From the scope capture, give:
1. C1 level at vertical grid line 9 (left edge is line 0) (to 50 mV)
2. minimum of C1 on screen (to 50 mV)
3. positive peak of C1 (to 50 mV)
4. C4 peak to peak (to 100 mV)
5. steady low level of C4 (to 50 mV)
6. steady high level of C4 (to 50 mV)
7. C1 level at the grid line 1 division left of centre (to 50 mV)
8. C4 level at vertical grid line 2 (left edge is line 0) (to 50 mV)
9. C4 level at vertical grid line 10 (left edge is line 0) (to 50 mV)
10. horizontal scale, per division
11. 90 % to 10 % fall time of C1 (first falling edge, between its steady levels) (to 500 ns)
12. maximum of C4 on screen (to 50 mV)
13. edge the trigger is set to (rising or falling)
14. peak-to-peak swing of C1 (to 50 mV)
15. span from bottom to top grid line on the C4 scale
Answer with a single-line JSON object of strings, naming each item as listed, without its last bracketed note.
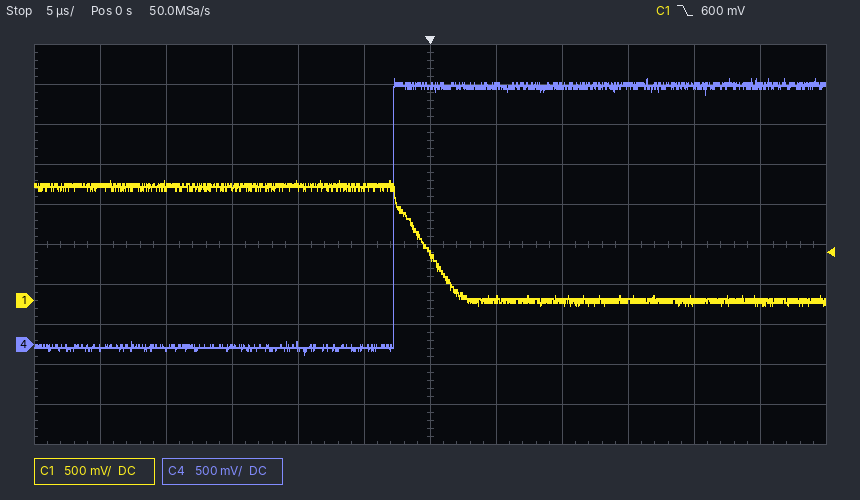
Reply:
{"C1 level at vertical grid line 9 (left edge is line 0)": "0 mV", "minimum of C1 on screen": "-50 mV", "positive peak of C1": "1.50 V", "C4 peak to peak": "3.40 V", "steady low level of C4": "-50 mV", "steady high level of C4": "3.25 V", "C1 level at the grid line 1 division left of centre": "1.40 V", "C4 level at vertical grid line 2 (left edge is line 0)": "-50 mV", "C4 level at vertical grid line 10 (left edge is line 0)": "3.25 V", "horizontal scale, per division": "5 µs", "90 % to 10 % fall time of C1 (first falling edge, between its steady levels)": "4.5 µs", "maximum of C4 on screen": "3.30 V", "edge the trigger is set to": "falling", "peak-to-peak swing of C1": "1.55 V", "span from bottom to top grid line on the C4 scale": "5 V"}
